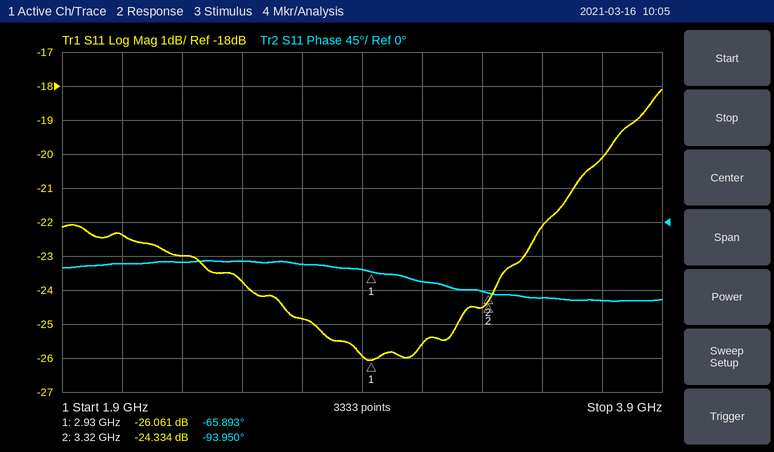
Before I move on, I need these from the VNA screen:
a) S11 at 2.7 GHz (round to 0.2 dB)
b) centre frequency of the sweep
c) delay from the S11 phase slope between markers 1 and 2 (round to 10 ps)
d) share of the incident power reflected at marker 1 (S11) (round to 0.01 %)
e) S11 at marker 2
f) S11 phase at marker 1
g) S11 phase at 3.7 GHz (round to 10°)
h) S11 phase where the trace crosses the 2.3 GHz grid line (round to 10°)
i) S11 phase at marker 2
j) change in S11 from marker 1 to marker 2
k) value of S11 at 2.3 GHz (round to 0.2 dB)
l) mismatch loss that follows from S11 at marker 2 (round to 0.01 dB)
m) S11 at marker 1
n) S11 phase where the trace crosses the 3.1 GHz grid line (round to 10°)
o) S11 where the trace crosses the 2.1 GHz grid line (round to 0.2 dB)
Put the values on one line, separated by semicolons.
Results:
-24.8 dB; 2.9 GHz; 200 ps; 0.25 %; -24.334 dB; -65.893°; -100°; -50°; -93.950°; 1.727 dB; -23.0 dB; 0.02 dB; -26.061 dB; -80°; -22.4 dB
